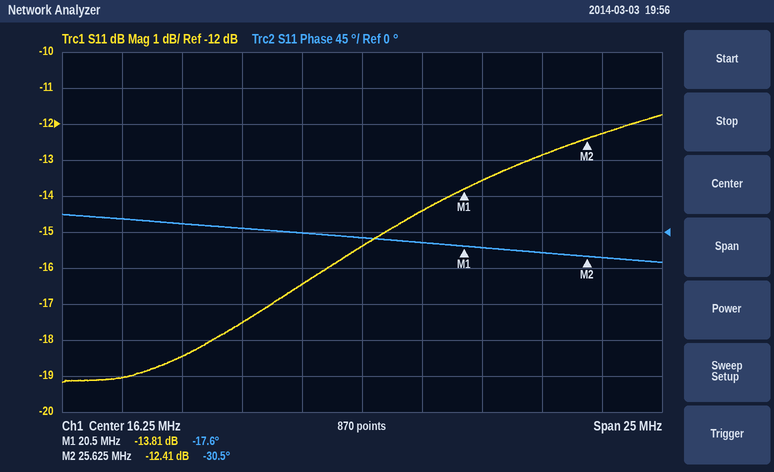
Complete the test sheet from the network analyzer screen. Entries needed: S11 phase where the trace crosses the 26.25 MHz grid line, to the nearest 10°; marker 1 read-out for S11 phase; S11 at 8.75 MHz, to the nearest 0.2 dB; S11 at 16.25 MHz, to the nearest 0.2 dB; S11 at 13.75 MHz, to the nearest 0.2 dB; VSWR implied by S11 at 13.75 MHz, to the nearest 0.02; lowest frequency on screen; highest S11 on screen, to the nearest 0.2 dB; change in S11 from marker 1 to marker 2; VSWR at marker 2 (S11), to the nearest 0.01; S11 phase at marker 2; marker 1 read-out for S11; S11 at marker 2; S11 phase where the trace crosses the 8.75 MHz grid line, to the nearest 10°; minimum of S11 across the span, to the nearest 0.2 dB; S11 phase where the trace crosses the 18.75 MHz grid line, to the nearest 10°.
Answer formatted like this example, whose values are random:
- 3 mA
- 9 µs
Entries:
- -30°
- -17.6°
- -18.4 dB
- -15.4 dB
- -16.4 dB
- 1.36
- 3.75 MHz
- -11.8 dB
- 1.40 dB
- 1.63
- -30.5°
- -13.81 dB
- -12.41 dB
- 10°
- -19.2 dB
- -10°
